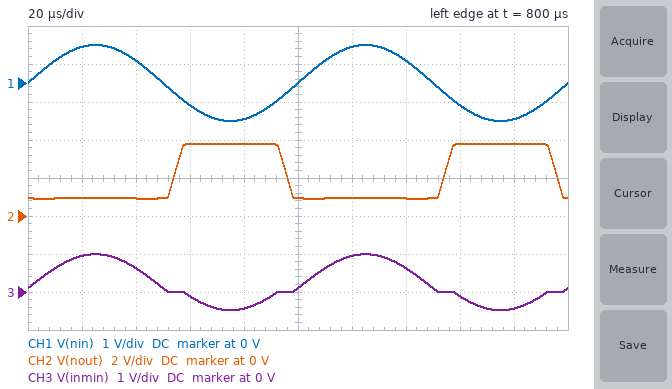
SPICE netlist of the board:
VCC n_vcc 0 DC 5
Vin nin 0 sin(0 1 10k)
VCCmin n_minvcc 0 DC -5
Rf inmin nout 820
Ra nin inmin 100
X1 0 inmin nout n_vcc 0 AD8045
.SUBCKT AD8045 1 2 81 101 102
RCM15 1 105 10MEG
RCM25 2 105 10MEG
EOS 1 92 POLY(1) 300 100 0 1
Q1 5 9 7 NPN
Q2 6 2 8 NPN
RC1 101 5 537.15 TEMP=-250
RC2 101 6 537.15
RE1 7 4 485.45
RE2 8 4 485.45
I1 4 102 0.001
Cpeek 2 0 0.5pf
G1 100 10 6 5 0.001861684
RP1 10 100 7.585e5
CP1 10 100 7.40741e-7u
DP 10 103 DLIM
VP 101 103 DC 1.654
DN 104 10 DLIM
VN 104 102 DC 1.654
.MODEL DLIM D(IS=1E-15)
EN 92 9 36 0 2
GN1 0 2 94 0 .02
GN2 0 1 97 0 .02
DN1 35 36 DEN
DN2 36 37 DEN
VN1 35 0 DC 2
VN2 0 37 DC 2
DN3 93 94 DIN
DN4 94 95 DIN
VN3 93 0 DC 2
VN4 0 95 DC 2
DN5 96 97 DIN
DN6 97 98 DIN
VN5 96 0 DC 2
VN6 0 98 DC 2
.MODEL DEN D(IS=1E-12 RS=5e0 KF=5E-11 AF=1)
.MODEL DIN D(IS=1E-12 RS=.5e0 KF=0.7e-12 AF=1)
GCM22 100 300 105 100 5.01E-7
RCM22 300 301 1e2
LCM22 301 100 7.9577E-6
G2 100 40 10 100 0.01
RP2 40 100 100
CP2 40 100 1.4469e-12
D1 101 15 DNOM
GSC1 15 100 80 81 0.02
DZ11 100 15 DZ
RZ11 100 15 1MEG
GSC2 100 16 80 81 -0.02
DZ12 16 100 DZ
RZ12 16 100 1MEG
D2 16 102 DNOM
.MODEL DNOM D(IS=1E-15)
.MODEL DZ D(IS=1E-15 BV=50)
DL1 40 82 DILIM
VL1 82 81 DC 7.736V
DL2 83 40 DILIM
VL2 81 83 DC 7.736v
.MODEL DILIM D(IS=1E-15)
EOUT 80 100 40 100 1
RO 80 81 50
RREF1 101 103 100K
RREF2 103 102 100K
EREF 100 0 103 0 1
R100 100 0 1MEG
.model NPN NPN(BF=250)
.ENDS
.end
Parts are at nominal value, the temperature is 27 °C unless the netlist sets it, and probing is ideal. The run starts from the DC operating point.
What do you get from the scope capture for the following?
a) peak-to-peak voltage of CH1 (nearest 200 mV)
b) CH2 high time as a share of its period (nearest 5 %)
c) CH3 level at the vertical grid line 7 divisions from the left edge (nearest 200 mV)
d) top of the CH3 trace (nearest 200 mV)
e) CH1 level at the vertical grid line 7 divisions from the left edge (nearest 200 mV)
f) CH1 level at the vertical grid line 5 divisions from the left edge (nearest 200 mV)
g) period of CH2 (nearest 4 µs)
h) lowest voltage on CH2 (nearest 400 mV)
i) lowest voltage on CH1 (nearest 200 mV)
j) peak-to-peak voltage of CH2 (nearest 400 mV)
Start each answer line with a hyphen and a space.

- 2.0 V
- 40 %
- 600 mV
- 1.0 V
- 600 mV
- 0 V
- 100 µs
- 800 mV
- -1.0 V
- 2.8 V
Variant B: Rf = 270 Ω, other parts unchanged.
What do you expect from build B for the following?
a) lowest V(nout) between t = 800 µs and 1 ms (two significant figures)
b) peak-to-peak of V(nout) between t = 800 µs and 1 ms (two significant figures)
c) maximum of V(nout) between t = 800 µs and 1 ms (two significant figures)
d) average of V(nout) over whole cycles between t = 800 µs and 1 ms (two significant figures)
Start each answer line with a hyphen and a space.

- 840 mV
- 1.9 V
- 2.7 V
- 1.4 V
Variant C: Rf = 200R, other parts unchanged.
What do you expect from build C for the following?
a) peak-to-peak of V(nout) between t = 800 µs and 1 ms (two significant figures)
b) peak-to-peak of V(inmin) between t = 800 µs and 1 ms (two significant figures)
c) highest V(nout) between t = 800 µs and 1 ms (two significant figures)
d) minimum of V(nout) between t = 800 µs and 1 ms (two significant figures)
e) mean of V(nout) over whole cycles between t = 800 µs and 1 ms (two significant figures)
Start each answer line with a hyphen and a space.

- 1.2 V
- 980 mV
- 2.0 V
- 810 mV
- 1.1 V
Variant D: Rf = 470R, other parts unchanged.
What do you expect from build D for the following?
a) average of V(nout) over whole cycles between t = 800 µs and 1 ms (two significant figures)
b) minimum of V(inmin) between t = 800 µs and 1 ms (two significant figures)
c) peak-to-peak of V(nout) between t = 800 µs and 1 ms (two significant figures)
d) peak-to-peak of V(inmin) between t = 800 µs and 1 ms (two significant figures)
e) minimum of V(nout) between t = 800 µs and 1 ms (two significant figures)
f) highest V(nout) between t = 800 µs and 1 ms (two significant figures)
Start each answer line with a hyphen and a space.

- 1.8 V
- -190 mV
- 2.7 V
- 1.2 V
- 890 mV
- 3.6 V
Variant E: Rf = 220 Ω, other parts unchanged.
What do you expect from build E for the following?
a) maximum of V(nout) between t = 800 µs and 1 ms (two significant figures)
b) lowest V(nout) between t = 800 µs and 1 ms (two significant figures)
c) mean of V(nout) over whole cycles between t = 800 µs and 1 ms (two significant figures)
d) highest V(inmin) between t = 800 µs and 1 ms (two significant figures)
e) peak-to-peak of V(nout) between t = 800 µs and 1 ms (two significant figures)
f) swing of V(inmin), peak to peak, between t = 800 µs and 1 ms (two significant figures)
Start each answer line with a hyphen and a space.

- 2.2 V
- 820 mV
- 1.2 V
- 980 mV
- 1.4 V
- 980 mV
